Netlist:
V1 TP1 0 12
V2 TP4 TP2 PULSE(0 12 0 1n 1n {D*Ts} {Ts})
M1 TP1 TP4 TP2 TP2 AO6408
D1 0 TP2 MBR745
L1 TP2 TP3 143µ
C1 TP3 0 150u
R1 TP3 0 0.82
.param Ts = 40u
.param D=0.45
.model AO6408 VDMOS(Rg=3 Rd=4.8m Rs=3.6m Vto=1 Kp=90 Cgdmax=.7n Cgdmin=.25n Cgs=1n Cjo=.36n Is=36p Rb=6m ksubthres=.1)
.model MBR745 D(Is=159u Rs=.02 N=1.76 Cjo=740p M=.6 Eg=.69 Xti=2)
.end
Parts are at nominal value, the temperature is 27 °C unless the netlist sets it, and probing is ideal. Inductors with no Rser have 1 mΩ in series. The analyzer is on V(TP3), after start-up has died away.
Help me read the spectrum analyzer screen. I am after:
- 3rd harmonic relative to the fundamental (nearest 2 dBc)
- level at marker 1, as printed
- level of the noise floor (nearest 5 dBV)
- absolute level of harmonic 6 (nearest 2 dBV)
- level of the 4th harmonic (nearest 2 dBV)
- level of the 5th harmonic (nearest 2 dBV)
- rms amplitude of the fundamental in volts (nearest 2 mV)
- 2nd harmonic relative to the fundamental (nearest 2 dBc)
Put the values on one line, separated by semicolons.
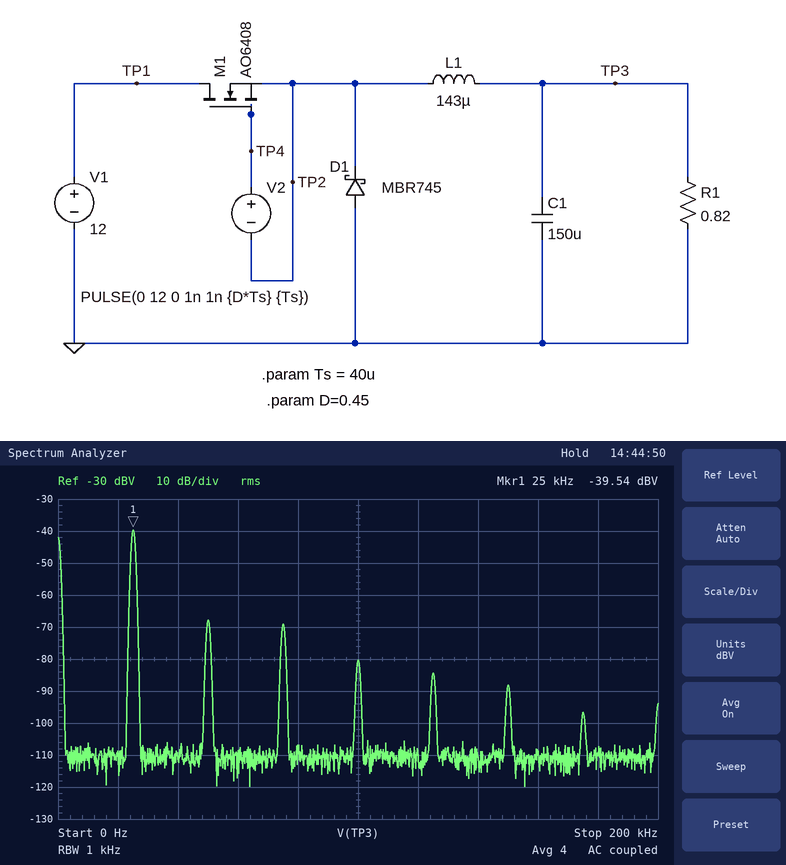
-30 dBc; -39.54 dBV; -110 dBV; -88 dBV; -80 dBV; -84 dBV; 10 mV; -28 dBc
